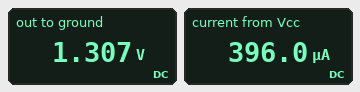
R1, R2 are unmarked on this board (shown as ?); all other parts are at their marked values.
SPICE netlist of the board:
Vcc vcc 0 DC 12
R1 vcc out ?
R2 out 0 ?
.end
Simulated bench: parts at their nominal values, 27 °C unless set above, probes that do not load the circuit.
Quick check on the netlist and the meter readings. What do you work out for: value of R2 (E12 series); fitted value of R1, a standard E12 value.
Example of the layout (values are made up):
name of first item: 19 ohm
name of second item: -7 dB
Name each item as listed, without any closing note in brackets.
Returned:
value of R2: 3.3 kΩ
fitted value of R1, a standard E12 value: 27 kΩ
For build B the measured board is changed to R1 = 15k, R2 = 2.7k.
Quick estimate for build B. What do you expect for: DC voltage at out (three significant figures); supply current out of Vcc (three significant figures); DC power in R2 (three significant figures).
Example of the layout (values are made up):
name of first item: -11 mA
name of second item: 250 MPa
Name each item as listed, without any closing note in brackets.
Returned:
DC voltage at out: 1.83 V
supply current out of Vcc: 678 µA
DC power in R2: 1.24 mW
